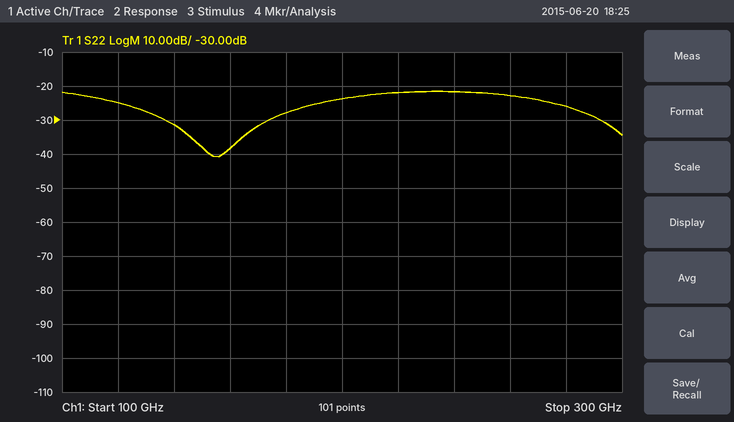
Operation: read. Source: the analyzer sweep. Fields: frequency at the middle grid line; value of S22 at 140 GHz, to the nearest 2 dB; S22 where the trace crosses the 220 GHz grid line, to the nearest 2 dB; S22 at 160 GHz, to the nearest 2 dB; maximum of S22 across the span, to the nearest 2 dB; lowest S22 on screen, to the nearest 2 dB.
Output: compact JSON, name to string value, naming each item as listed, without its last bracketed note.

{"frequency at the middle grid line": "200 GHz", "value of S22 at 140 GHz, to the nearest 2 dB": "-32 dB", "S22 where the trace crosses the 220 GHz grid line, to the nearest 2 dB": "-22 dB", "S22 at 160 GHz, to the nearest 2 dB": "-38 dB", "maximum of S22 across the span, to the nearest 2 dB": "-22 dB", "lowest S22 on screen, to the nearest 2 dB": "-40 dB"}
